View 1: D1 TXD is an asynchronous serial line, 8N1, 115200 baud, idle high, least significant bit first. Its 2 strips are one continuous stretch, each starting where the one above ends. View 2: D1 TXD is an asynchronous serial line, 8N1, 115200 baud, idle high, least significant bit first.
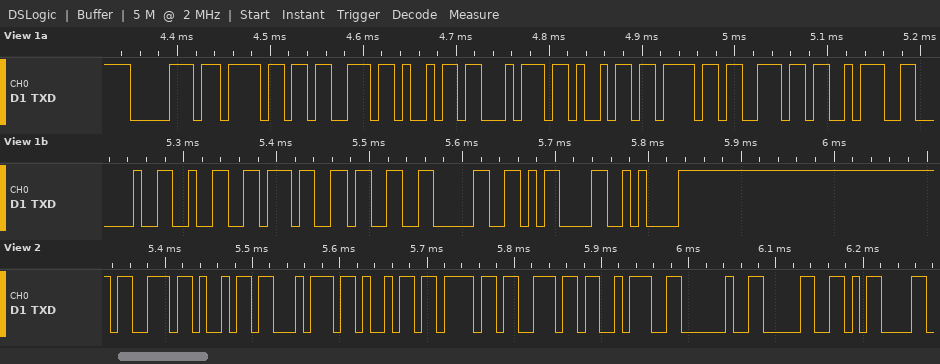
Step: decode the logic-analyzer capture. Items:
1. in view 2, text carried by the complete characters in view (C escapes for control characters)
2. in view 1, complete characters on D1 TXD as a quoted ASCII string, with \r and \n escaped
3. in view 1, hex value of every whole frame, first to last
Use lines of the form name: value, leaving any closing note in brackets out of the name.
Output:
in view 2, text carried by the complete characters in view: "sition: 0\r"
in view 1, complete characters on D1 TXD as a quoted ASCII string, with \r and \n escaped: "position: 2730\r\n"
in view 1, hex value of every whole frame, first to last: 70 6F 73 69 74 69 6F 6E 3A 20 32 37 33 30 0D 0A
